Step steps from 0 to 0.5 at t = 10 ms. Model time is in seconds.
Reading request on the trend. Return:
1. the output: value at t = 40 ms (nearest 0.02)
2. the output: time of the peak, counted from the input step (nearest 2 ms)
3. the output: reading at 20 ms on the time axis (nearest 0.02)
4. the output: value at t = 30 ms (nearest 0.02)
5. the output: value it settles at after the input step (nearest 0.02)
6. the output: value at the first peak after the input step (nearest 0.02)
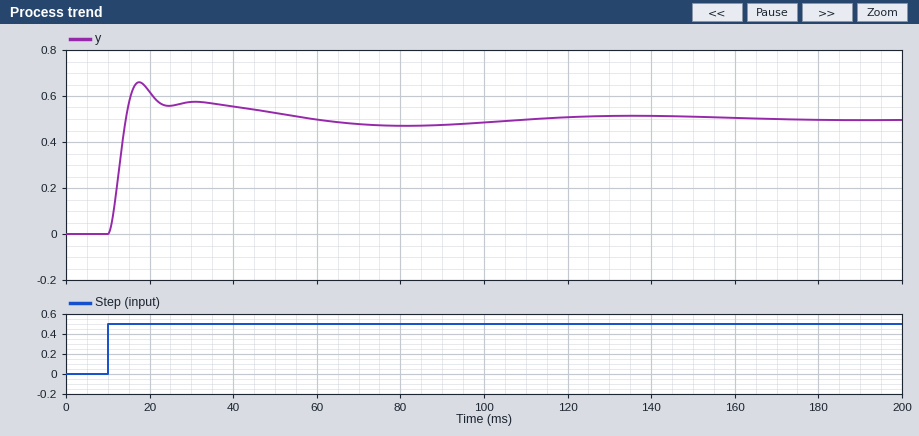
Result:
0.56
8 ms
0.62
0.58
0.50
0.66
